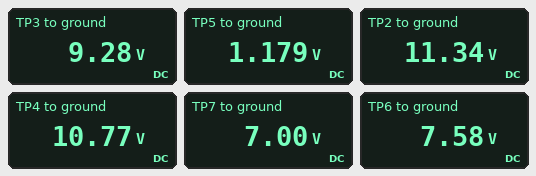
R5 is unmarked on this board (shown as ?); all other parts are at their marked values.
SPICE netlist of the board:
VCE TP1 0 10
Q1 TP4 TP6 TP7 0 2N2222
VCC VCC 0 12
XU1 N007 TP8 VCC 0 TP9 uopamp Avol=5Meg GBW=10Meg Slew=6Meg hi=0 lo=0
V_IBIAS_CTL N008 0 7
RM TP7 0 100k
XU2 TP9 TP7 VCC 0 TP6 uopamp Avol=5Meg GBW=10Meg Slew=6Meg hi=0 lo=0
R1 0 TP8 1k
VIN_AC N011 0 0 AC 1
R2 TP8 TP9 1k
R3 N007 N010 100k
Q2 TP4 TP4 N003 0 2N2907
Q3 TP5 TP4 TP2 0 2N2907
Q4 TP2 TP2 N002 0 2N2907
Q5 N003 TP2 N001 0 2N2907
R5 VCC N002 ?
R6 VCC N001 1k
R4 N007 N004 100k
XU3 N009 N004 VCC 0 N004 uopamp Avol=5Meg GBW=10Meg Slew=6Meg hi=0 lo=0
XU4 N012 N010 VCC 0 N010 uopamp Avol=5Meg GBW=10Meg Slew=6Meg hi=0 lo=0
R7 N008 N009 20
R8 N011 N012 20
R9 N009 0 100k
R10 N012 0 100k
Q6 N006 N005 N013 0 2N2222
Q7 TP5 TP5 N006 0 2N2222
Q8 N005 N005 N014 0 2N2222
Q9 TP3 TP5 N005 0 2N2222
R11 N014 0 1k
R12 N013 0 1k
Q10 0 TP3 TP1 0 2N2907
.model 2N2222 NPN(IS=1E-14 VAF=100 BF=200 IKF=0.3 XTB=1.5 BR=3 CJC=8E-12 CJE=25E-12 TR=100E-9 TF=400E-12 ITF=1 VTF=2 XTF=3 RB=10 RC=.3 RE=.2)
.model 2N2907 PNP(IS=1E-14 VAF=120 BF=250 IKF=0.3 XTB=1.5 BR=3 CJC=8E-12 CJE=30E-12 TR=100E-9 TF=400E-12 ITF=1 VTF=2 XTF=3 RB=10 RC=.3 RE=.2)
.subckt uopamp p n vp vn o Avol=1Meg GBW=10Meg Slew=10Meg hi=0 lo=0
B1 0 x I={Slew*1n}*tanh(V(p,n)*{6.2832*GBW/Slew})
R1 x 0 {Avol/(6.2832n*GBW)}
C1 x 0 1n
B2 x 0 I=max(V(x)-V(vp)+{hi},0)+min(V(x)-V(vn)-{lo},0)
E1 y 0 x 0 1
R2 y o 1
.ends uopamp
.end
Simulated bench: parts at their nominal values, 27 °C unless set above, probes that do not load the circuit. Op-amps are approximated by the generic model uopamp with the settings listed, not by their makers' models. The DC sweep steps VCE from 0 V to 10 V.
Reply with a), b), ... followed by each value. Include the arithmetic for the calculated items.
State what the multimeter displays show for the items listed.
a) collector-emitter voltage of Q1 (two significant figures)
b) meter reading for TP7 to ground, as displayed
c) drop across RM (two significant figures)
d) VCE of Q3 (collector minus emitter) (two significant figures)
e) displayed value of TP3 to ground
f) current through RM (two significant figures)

a) 10.77 V - 7 V = 3.8 V
b) 7.00 V
c) 7 V = 7.0 V
d) 1.179 V - 11.34 V = -10 V
e) 9.28 V
f) (7 V) / 100 kΩ = 70 µA
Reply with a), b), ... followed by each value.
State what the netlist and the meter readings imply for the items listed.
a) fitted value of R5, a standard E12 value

a) 2.2 kΩ
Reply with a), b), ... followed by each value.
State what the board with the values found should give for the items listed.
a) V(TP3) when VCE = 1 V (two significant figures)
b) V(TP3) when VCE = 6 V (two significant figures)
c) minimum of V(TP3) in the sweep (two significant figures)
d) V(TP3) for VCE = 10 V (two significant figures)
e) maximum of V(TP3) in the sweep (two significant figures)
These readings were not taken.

a) 580 mV
b) 5.3 V
c) 580 mV
d) 9.3 V
e) 9.3 V
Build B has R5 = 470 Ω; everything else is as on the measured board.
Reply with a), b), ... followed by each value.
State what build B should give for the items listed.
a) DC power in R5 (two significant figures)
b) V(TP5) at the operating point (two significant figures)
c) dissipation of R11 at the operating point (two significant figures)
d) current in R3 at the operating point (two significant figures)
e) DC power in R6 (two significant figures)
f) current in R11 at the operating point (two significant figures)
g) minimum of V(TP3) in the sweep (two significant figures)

a) 6.6 µW
b) 1.3 V
c) 14 µW
d) 35 µA
e) 4.8 µW
f) 120 µA
g) 650 mV
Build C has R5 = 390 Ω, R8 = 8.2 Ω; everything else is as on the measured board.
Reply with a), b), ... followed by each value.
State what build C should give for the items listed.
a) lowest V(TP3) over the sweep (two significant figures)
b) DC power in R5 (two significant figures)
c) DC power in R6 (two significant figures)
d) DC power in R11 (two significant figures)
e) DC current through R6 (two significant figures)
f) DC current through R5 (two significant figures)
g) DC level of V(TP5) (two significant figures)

a) 660 mV
b) 7.0 µW
c) 4.8 µW
d) 18 µW
e) 69 µA
f) 130 µA
g) 1.3 V
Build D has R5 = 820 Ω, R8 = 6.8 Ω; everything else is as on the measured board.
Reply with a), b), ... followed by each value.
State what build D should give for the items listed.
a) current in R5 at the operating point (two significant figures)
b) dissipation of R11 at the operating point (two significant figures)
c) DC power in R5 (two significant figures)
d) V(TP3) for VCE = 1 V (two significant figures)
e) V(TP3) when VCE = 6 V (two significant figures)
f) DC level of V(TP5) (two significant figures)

a) 80 µA
b) 6.5 µW
c) 5.3 µW
d) 620 mV
e) 5.3 V
f) 1.3 V
